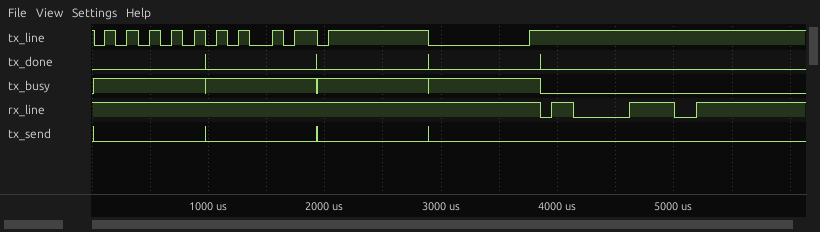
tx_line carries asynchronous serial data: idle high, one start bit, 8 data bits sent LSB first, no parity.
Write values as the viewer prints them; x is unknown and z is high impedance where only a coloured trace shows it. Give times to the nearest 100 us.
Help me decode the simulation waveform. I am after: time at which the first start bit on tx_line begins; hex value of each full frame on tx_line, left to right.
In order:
0 us
55, A5, FF, 00
